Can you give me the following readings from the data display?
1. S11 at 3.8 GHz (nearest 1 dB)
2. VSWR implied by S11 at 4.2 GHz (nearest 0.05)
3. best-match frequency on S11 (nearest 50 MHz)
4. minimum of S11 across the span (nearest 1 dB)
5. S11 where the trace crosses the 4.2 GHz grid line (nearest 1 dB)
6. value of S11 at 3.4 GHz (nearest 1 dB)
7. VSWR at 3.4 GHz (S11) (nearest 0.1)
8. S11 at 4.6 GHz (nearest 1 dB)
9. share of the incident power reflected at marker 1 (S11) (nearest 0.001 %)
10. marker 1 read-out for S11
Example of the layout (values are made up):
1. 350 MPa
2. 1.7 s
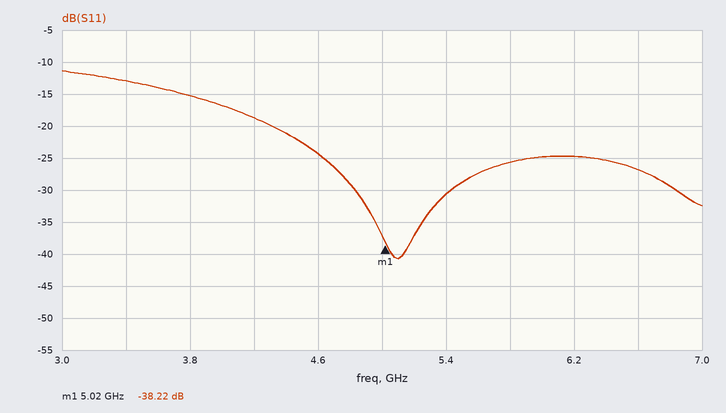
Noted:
1. -15 dB
2. 1.25
3. 5.10 GHz
4. -41 dB
5. -19 dB
6. -13 dB
7. 1.6
8. -24 dB
9. 0.015 %
10. -38.22 dB
